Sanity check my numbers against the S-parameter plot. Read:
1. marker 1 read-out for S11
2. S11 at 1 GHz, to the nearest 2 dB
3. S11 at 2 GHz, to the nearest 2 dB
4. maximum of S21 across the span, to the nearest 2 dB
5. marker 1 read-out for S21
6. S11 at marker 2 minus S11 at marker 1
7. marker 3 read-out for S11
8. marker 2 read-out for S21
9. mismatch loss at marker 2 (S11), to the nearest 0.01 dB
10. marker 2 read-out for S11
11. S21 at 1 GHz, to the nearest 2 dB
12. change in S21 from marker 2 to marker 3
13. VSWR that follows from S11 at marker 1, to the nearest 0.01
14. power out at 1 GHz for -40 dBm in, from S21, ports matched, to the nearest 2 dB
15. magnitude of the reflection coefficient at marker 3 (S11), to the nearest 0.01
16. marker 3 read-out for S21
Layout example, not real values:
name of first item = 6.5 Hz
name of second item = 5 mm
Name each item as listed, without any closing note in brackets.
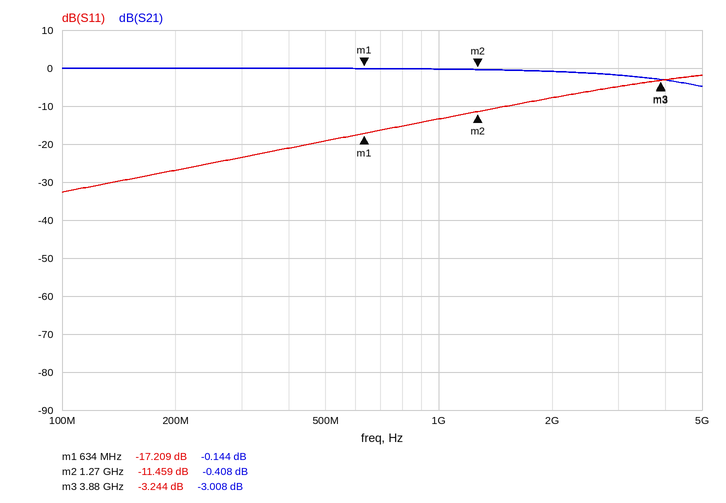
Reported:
marker 1 read-out for S11 = -17.209 dB
S11 at 1 GHz, to the nearest 2 dB = -14 dB
S11 at 2 GHz, to the nearest 2 dB = -8 dB
maximum of S21 across the span, to the nearest 2 dB = 0 dB
marker 1 read-out for S21 = -0.144 dB
S11 at marker 2 minus S11 at marker 1 = 5.750 dB
marker 3 read-out for S11 = -3.244 dB
marker 2 read-out for S21 = -0.408 dB
mismatch loss at marker 2 (S11), to the nearest 0.01 dB = 0.32 dB
marker 2 read-out for S11 = -11.459 dB
S21 at 1 GHz, to the nearest 2 dB = 0 dB
change in S21 from marker 2 to marker 3 = -2.600 dB
VSWR that follows from S11 at marker 1, to the nearest 0.01 = 1.32
power out at 1 GHz for -40 dBm in, from S21, ports matched, to the nearest 2 dB = -40 dBm
magnitude of the reflection coefficient at marker 3 (S11), to the nearest 0.01 = 0.69
marker 3 read-out for S21 = -3.008 dB
